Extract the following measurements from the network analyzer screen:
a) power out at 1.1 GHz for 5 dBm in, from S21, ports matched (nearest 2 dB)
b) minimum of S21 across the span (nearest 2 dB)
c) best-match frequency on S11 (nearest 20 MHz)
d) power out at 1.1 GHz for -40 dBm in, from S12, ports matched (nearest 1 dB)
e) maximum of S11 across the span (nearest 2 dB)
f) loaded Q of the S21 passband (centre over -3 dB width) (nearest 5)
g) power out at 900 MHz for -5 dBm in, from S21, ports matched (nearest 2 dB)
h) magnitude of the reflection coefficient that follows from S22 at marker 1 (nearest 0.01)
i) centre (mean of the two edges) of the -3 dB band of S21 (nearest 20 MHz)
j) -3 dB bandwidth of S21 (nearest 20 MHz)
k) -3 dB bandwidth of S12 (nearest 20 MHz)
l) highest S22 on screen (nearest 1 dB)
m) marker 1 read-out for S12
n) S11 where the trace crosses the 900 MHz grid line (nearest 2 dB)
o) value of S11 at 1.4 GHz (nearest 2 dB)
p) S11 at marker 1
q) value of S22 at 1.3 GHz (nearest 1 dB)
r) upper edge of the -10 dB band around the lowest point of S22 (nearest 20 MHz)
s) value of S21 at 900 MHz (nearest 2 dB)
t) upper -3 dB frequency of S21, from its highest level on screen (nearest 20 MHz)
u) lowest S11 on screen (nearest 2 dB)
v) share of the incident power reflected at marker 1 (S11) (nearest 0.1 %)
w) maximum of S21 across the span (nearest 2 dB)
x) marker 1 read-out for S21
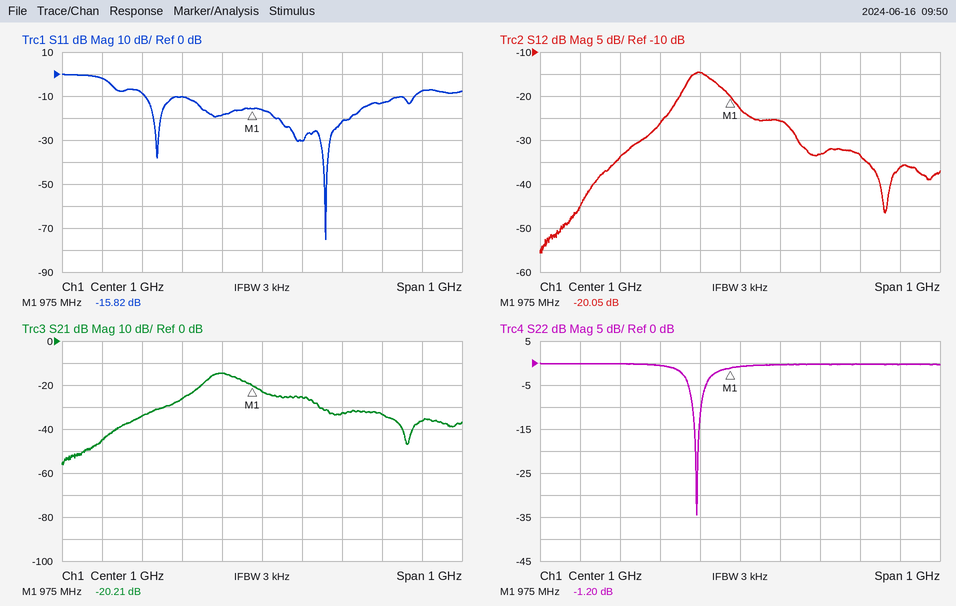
-20 dBm
-56 dB
1.16 GHz
-66 dBm
0 dB
10
-20 dBm
0.87
900 MHz
80 MHz
80 MHz
0 dB
-20.05 dB
-18 dB
-8 dB
-15.82 dB
0 dB
900 MHz
-14 dB
940 MHz
-76 dB
2.6 %
-14 dB
-20.21 dB
